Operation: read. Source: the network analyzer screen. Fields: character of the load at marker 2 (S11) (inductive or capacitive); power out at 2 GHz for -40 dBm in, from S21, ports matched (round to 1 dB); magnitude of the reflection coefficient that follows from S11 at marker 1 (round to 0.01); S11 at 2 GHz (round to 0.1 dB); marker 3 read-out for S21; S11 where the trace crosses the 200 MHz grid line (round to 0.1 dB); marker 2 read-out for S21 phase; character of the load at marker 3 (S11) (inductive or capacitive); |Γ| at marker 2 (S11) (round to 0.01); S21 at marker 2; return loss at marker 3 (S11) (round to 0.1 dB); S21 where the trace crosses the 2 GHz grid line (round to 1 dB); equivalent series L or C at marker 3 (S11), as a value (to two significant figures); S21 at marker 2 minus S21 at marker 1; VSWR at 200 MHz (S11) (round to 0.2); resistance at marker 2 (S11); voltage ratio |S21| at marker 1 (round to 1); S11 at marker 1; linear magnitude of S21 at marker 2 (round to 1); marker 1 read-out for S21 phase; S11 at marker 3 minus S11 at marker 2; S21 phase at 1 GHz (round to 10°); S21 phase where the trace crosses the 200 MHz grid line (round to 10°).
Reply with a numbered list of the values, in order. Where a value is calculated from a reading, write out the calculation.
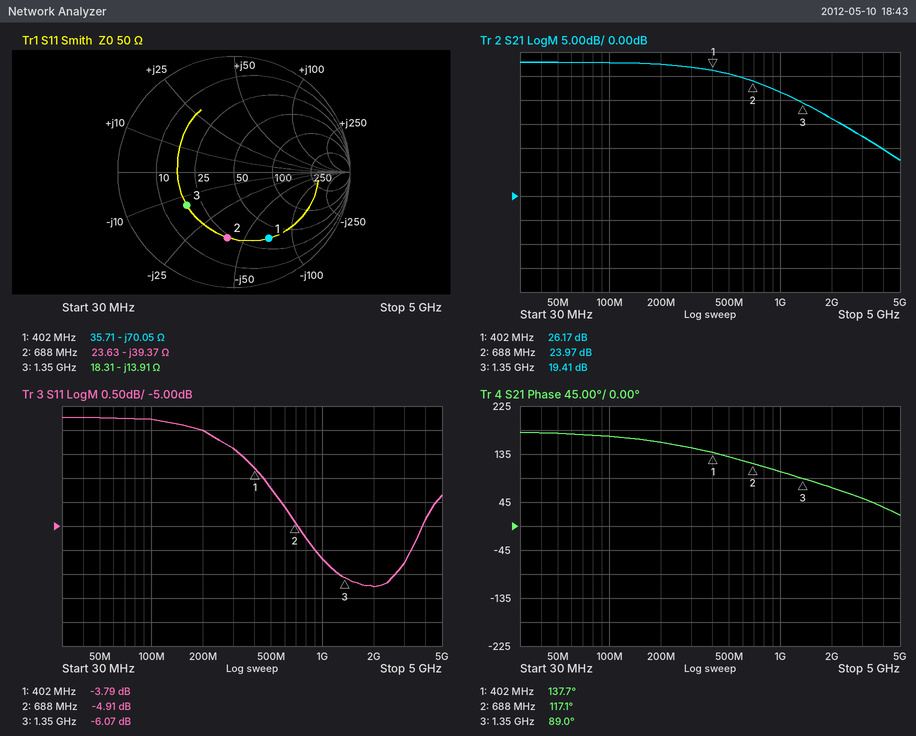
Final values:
1. capacitive
2. -40 dBm + (16 dB) = -24 dBm
3. 10^(-3.79/20) ≈ 0.65
4. -6.3 dB
5. 19.41 dB
6. -3.0 dB
7. 117.1°
8. capacitive
9. 0.57
10. 23.97 dB
11. 6.1 dB
12. 16 dB
13. C = 1/(2π × 1.35 GHz × 13.91 Ω) ≈ 8.5 pF
14. 23.97 − (26.17) = -2.20 dB
15. |Γ| = 10^(-3/20) = 0.7079; VSWR = (1 + 0.7079)/(1 − 0.7079) ≈ 5.8
16. 23.63 Ω
17. 10^(26.17/20) ≈ 20
18. -3.79 dB
19. 10^(23.97/20) ≈ 16
20. 137.7°
21. -6.07 − (-4.91) = -1.16 dB
22. 100°
23. 160°
